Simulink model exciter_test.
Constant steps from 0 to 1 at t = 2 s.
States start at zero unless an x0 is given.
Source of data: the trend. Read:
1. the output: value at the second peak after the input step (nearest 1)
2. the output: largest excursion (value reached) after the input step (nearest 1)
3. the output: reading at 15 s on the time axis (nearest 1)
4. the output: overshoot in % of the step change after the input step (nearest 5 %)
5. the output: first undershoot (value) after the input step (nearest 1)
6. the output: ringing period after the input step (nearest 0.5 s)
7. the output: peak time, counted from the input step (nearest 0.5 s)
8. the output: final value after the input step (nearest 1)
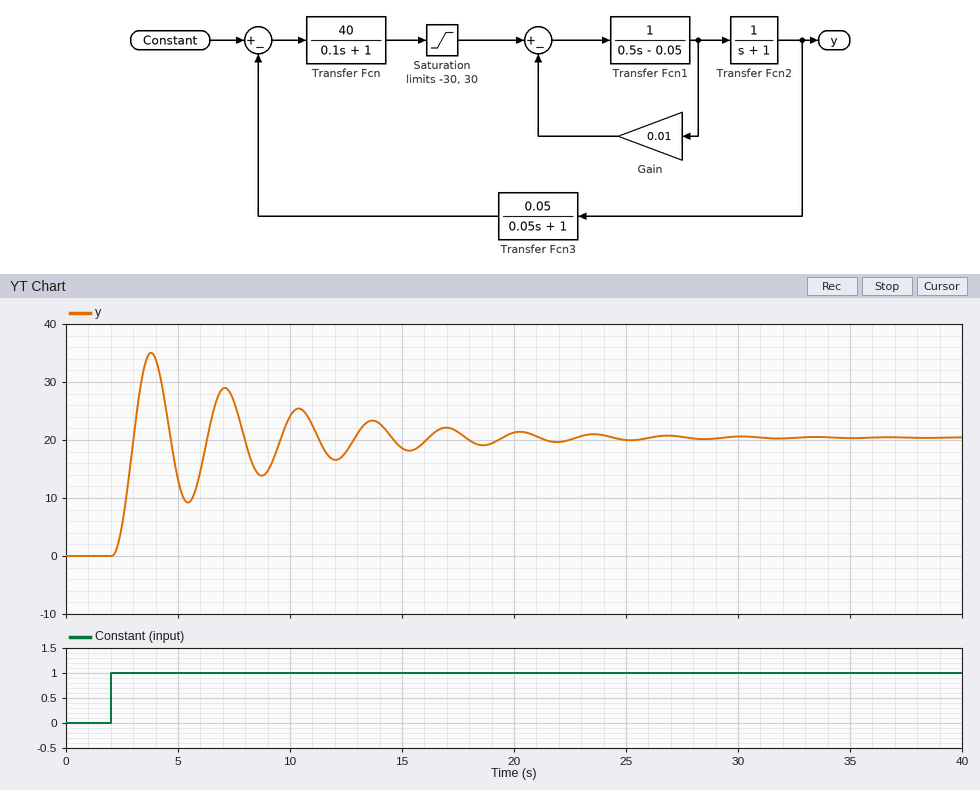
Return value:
29
35
19
70 %
9
3.5 s
2.0 s
20
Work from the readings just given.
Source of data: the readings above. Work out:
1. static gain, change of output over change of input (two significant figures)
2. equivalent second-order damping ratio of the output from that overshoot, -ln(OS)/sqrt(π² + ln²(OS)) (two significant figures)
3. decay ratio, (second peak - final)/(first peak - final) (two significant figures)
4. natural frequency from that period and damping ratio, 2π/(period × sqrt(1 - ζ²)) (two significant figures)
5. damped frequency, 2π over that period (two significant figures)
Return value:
20
0.11
0.60
1.8 rad/s
1.8 rad/s
